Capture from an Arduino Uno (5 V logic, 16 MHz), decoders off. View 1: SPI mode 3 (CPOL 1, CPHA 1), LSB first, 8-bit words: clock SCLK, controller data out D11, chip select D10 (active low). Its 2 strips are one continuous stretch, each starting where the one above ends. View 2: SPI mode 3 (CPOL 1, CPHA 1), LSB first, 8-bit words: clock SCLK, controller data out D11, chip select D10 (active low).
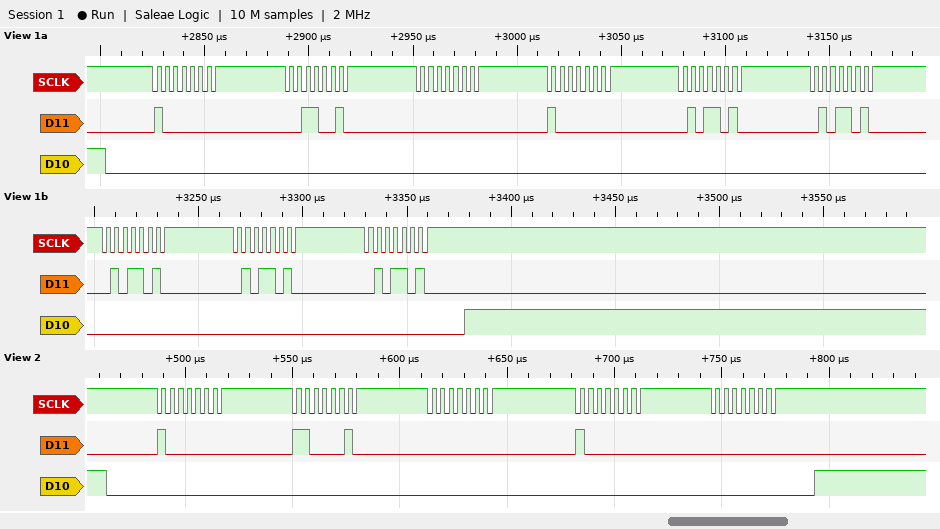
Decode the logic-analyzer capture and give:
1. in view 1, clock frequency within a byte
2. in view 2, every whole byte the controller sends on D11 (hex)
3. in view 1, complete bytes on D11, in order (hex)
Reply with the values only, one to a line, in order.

250 kHz
0x01 0x43 0x00 0x01 0x00
0x01 0x4C 0x00 0x01 0x5A 0x5A 0x5A 0x5A 0x5A
